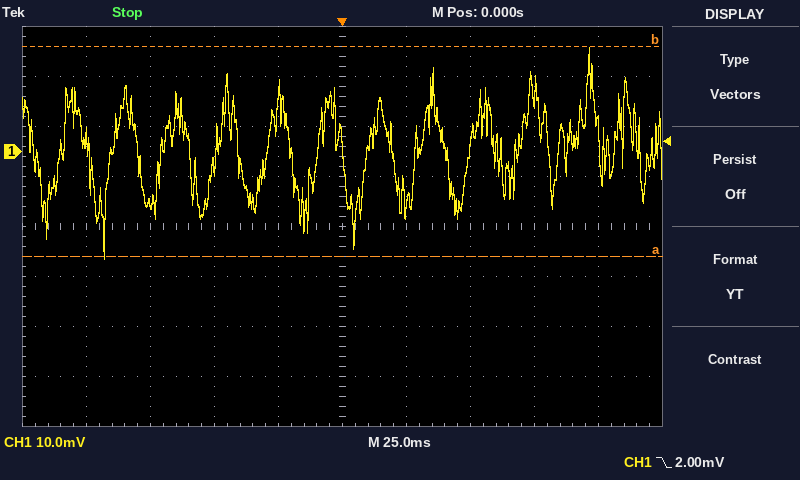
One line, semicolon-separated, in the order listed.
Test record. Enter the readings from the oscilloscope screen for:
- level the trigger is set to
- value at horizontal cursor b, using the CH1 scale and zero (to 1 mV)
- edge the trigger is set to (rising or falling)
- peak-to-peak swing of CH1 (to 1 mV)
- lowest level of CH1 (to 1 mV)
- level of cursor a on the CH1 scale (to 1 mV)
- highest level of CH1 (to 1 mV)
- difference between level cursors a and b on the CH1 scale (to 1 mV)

2.00 mV; 21 mV; falling; 42 mV; -21 mV; -21 mV; 21 mV; 42 mV
